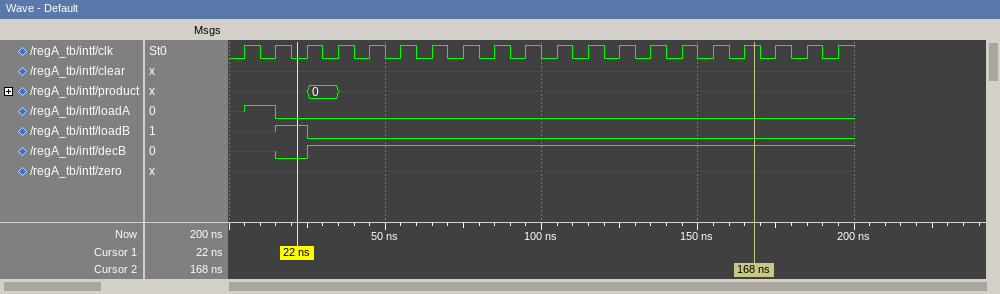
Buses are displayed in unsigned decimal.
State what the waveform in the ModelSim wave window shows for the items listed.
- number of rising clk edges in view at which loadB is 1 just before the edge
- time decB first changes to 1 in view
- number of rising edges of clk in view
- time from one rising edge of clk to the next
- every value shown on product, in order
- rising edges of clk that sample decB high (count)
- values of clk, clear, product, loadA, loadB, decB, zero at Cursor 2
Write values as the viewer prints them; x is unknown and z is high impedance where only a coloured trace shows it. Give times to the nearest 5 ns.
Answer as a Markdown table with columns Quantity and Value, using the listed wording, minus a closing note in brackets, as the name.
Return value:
| Quantity | Value |
|---|---|
| number of rising clk edges in view at which loadB is 1 just before the edge | 1 |
| time decB first changes to 1 in view | 25 ns |
| number of rising edges of clk in view | 20 |
| time from one rising edge of clk to the next | 10 ns |
| every value shown on product, in order | x, 0, x |
| rising edges of clk that sample decB high | 17 |
| values of clk, clear, product, loadA, loadB, decB, zero at Cursor 2 | clk=1, clear=x, product=x, loadA=0, loadB=0, decB=1, zero=x |
